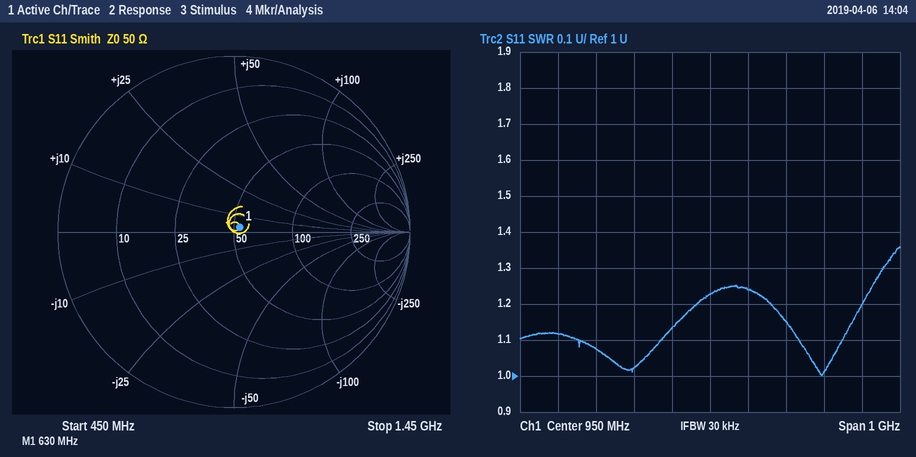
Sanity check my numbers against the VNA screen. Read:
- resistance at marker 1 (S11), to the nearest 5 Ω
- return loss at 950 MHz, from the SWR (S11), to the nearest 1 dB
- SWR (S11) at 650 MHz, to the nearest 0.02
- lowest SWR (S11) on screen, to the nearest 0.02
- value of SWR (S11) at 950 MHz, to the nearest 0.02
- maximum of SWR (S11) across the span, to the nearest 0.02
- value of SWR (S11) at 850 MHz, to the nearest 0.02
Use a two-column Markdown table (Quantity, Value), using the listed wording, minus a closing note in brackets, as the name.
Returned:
| Quantity | Value |
|---|---|
| resistance at marker 1 (S11), to the nearest 5 Ω | 55 Ω |
| return loss at 950 MHz, from the SWR (S11), to the nearest 1 dB | 20 dB |
| SWR (S11) at 650 MHz, to the nearest 0.02 | 1.08 |
| lowest SWR (S11) on screen, to the nearest 0.02 | 1.00 |
| value of SWR (S11) at 950 MHz, to the nearest 0.02 | 1.22 |
| maximum of SWR (S11) across the span, to the nearest 0.02 | 1.36 |
| value of SWR (S11) at 850 MHz, to the nearest 0.02 | 1.14 |
